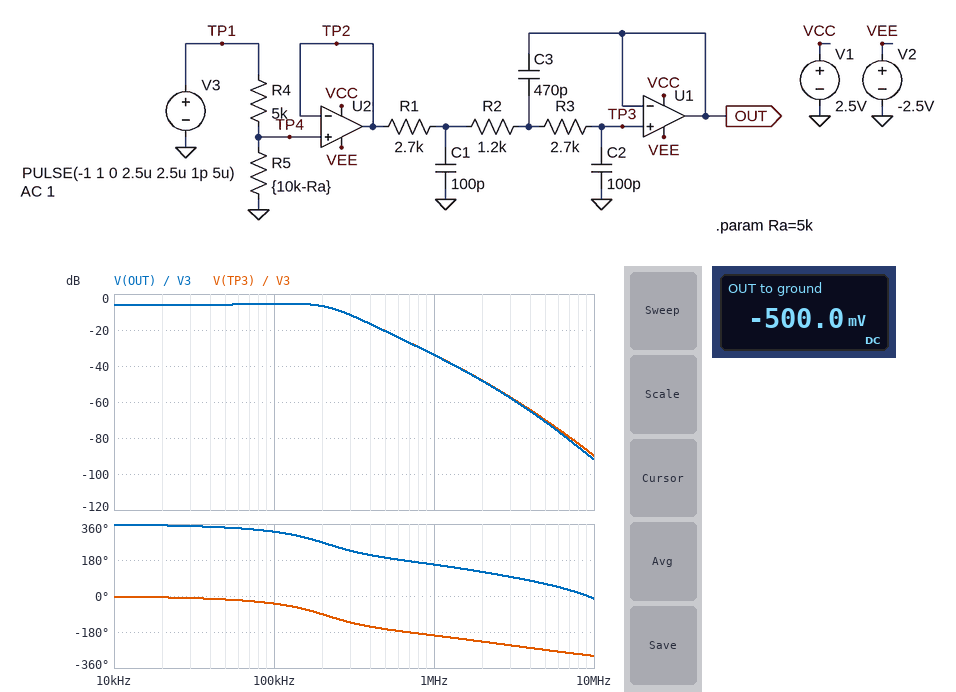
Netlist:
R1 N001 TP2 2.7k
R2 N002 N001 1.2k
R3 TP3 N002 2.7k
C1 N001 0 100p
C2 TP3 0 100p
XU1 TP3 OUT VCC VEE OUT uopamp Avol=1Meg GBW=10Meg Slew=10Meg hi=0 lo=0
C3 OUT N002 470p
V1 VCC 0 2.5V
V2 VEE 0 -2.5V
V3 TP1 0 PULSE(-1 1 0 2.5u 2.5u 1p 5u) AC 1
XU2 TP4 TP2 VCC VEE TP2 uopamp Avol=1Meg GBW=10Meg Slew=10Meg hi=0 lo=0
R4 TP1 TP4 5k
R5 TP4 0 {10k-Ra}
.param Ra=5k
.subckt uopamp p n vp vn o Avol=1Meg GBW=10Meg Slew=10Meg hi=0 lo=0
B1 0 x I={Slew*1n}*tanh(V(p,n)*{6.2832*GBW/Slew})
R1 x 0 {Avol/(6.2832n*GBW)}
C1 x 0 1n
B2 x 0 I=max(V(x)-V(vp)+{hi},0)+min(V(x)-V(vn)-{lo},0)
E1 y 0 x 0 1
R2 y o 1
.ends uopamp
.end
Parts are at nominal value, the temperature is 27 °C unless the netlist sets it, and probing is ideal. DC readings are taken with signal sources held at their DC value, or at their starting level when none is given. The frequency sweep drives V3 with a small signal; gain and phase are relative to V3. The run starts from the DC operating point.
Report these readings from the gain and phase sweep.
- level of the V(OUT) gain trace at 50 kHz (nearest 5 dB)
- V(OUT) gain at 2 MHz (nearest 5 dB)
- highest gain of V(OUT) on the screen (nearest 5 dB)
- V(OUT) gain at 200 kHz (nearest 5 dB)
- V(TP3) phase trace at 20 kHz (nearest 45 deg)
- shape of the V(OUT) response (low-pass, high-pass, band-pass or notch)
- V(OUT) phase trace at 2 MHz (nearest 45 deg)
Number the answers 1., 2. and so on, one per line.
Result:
1. -5 dB
2. -50 dB
3. -5 dB
4. -5 dB
5. 0 deg
6. low-pass
7. 135 deg
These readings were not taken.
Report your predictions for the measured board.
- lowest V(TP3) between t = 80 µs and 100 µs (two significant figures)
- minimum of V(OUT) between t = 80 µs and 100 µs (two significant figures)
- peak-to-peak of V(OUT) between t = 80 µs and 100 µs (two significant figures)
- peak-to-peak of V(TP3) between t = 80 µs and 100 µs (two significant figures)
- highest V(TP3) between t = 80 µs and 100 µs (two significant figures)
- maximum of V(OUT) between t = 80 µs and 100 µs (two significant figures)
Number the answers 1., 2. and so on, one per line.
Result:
1. -370 mV
2. -370 mV
3. 750 mV
4. 750 mV
5. 370 mV
6. 370 mV
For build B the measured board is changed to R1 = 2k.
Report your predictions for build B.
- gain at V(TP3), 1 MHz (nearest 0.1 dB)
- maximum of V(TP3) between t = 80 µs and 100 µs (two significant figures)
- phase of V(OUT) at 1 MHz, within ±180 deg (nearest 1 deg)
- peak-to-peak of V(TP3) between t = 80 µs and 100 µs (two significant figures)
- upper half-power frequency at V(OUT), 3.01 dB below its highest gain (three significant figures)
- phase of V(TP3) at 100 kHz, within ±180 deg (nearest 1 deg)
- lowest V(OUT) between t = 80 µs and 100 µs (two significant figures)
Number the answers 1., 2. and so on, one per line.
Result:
1. -31.8 dB
2. 430 mV
3. 160 deg
4. 860 mV
5. 271 kHz
6. -32 deg
7. -430 mV
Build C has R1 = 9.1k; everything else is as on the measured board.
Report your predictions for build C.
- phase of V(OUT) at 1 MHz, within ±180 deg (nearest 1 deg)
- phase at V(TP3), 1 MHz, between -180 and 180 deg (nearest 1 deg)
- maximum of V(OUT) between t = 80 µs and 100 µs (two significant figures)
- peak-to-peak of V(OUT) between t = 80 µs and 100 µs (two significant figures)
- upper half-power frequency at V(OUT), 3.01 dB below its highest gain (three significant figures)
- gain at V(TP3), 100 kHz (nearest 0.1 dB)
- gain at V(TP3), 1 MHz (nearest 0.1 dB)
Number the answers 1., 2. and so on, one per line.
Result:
1. 150 deg
2. 156 deg
3. 130 mV
4. 260 mV
5. 103 kHz
6. -8.9 dB
7. -43.1 dB
